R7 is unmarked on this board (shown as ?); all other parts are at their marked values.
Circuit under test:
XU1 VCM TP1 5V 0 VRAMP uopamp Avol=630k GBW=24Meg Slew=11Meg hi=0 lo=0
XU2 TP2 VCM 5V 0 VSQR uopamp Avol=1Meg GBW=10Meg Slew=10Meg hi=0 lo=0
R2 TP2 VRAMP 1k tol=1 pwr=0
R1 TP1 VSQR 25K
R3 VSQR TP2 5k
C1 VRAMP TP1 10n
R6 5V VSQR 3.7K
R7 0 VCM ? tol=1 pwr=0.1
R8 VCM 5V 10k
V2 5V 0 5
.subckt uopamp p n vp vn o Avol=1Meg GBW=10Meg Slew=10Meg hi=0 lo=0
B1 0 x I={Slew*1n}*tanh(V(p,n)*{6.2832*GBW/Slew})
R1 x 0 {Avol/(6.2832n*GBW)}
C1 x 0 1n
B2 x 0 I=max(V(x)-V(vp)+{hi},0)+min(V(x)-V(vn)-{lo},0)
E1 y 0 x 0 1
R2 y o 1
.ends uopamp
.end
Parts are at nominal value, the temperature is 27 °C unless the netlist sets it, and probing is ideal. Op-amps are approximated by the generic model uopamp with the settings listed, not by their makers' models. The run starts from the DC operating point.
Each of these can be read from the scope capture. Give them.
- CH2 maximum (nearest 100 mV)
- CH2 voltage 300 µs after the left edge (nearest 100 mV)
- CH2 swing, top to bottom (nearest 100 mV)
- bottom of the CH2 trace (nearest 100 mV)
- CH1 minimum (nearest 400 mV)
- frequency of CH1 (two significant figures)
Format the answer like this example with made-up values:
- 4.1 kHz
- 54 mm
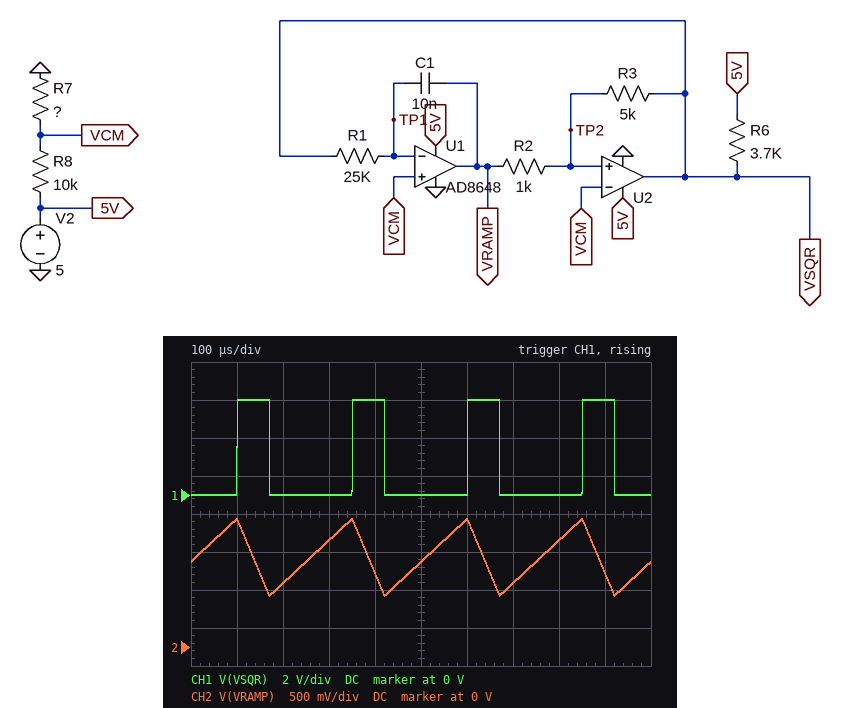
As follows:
- 1.7 V
- 1.4 V
- 1.0 V
- 700 mV
- 0 V
- 4.0 kHz
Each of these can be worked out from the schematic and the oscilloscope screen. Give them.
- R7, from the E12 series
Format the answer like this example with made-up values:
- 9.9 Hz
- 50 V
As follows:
- 3.9 kΩ
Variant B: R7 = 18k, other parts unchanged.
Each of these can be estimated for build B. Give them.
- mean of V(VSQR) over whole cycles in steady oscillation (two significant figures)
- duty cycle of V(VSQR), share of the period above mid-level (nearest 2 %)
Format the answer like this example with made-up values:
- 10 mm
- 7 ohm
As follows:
- 3.2 V
- 64 %
